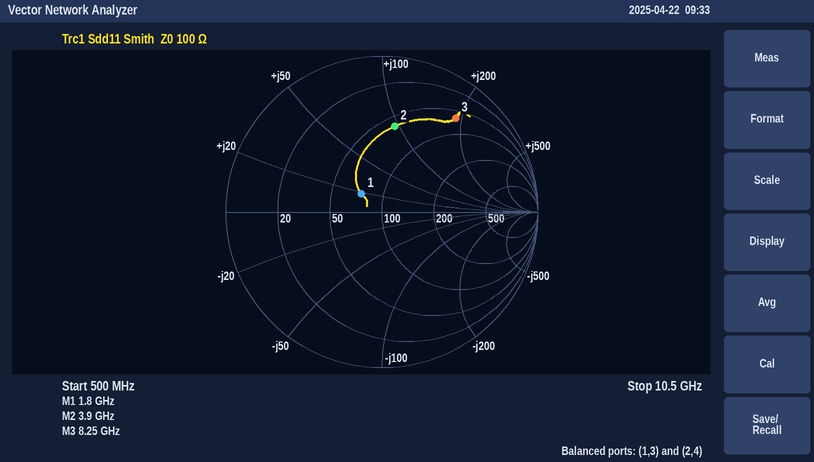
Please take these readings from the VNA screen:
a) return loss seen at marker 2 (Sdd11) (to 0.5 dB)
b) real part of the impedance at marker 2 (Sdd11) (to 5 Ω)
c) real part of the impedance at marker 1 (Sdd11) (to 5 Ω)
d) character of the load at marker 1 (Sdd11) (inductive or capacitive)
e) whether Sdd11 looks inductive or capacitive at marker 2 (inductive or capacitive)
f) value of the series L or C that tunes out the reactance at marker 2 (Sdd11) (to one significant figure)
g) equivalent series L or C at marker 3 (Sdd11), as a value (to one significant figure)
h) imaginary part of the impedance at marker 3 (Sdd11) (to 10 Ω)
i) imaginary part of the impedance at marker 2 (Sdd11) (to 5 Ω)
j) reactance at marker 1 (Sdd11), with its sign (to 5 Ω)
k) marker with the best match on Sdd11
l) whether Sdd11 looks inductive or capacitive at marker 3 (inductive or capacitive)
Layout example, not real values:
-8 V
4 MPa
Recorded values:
5.0 dB
60 Ω
75 Ω
inductive
inductive
400 fF
4 nH
+190 Ω
+95 Ω
+20 Ω
marker 1
inductive
